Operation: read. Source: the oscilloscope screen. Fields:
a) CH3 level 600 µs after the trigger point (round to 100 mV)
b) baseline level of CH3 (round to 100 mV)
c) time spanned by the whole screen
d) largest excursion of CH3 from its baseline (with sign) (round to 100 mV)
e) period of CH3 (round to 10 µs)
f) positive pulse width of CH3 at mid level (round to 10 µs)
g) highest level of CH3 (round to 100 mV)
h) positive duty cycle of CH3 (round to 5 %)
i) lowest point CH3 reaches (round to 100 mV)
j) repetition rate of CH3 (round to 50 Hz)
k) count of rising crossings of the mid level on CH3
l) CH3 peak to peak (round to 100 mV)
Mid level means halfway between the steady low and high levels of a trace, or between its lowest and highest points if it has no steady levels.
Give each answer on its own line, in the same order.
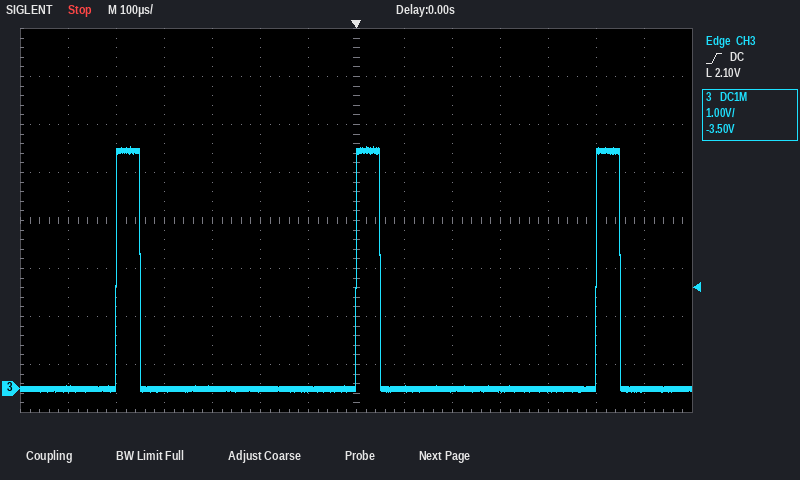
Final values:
0.0 V
0.0 V
1.4 ms
+5.0 V
500 µs
50 µs
5.0 V
10 %
-100 mV
2.00 kHz
3
5.1 V
